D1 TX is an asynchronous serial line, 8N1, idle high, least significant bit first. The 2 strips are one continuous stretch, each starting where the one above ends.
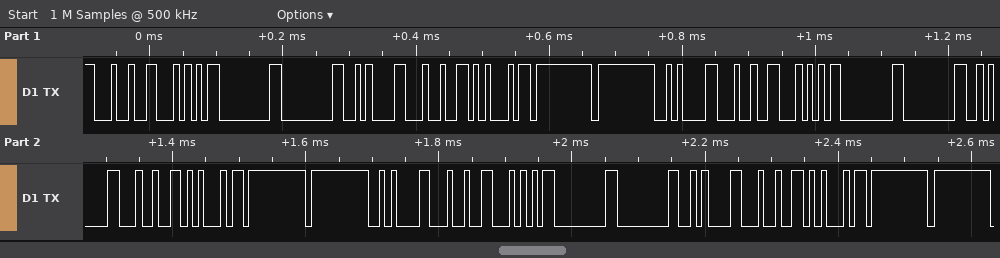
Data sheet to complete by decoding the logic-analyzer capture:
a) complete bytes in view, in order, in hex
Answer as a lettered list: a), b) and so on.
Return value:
a) 24 54 00 00 0A 24 45 FF FF 0A 24 54 00 00 0A 24 45 FF FF 0A 24 54 00 00 0A 24 45 FF FF
